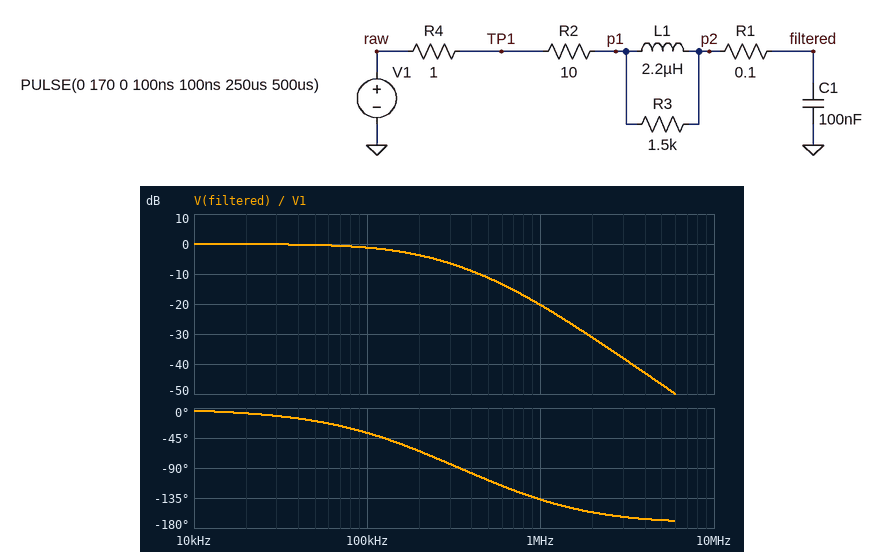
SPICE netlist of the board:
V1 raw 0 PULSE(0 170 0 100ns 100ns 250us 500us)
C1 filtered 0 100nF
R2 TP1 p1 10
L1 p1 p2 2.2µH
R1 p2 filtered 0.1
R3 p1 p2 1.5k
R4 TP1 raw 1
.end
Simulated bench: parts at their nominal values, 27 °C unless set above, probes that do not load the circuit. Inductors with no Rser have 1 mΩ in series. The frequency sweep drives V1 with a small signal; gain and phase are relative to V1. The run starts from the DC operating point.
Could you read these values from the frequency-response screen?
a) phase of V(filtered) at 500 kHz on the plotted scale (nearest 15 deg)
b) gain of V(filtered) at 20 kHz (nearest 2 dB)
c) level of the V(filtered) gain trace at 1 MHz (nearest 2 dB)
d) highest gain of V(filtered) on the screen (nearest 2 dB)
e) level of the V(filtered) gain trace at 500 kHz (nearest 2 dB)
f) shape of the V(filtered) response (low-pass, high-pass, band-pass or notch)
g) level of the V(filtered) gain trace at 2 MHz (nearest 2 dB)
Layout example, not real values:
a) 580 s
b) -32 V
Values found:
a) -105 deg
b) 0 dB
c) -20 dB
d) 0 dB
e) -12 dB
f) low-pass
g) -32 dB
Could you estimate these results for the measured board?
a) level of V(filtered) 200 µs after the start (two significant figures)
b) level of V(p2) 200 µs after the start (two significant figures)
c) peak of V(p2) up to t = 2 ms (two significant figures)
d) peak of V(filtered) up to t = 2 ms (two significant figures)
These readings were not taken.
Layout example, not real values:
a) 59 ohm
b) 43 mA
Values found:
a) 170 V
b) 170 V
c) 170 V
d) 170 V
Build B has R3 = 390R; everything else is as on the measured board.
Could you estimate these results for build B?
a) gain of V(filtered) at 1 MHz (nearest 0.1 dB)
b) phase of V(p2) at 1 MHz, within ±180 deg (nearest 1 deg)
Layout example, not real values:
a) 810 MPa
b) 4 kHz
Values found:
a) -20.5 dB
b) -133 deg
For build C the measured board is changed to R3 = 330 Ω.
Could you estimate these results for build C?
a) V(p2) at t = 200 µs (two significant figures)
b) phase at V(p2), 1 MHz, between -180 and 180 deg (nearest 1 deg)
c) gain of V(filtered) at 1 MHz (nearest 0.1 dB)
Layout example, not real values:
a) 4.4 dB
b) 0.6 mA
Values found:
a) 170 V
b) -133 deg
c) -20.5 dB
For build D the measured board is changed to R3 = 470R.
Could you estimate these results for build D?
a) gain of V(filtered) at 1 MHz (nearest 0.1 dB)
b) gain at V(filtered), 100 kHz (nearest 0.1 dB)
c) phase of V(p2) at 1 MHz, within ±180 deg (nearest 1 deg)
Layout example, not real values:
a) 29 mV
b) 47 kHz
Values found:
a) -20.5 dB
b) -1.2 dB
c) -133 deg
